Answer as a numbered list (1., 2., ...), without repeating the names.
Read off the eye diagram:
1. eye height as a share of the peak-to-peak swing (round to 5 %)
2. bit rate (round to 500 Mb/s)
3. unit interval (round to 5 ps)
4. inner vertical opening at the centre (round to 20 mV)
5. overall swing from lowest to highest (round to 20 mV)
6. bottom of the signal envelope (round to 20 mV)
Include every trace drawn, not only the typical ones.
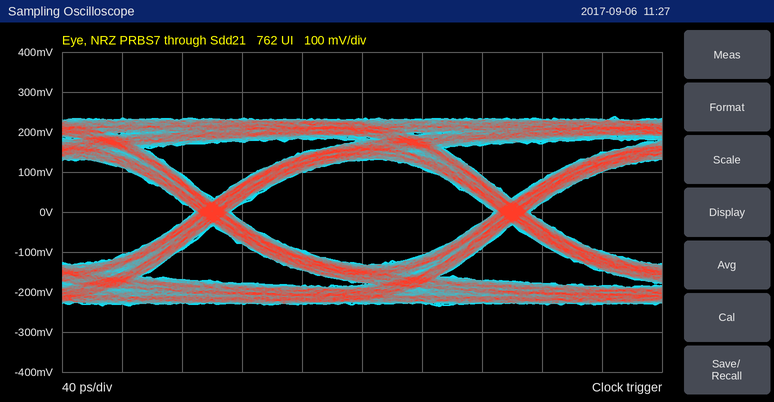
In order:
1. 55 %
2. 5.0 Gb/s
3. 200 ps
4. 260 mV
5. 480 mV
6. -240 mV
